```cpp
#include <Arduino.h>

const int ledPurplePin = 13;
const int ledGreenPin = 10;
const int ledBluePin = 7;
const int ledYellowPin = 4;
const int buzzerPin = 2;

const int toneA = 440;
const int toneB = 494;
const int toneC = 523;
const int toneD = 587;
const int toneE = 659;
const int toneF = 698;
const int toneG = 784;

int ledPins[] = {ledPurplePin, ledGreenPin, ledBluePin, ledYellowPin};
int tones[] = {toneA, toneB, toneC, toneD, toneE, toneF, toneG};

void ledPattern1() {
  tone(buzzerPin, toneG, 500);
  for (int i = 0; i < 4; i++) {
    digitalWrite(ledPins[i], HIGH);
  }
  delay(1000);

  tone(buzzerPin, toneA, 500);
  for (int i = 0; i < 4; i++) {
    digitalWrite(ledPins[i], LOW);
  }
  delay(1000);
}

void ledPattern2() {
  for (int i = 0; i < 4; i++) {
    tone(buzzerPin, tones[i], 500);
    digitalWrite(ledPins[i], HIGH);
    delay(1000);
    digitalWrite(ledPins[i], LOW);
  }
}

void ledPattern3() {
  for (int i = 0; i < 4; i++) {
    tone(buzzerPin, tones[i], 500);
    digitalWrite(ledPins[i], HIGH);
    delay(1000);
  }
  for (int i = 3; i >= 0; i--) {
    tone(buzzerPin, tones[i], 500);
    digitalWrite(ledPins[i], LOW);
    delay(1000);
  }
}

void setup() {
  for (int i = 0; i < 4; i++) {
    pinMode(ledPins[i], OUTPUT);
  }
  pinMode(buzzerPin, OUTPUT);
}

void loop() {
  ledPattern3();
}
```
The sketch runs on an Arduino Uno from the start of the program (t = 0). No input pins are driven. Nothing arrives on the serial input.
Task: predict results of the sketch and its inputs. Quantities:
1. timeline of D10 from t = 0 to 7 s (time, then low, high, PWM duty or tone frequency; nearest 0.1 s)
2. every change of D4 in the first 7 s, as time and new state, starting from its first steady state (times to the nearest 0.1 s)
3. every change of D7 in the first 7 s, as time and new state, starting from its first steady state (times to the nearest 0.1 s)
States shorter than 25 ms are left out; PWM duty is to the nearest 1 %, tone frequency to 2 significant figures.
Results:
0 s low; 1 s high; 6 s low
0 s low; 3 s high; 4 s low
0 s low; 2 s high; 5 s low
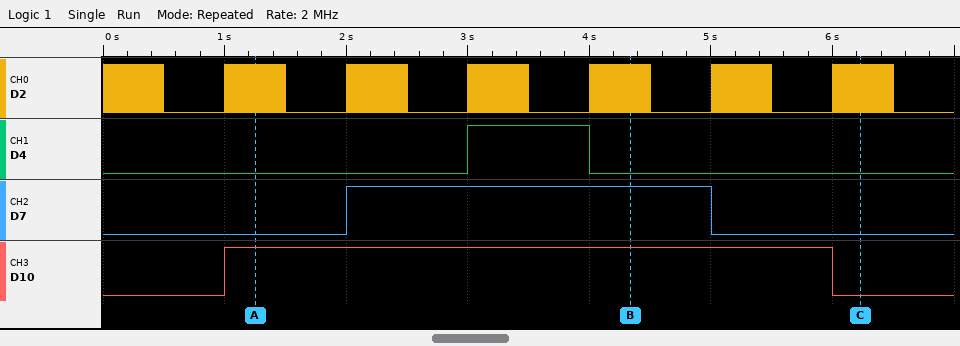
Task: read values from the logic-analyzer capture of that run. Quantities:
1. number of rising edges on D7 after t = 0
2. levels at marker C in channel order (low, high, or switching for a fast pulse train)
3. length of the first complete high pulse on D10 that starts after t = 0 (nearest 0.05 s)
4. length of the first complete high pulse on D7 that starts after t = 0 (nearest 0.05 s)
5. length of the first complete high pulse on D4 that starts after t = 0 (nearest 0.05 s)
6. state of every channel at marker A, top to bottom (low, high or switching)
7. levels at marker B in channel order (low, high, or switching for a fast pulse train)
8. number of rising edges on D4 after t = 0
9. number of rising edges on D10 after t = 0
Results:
1
D2 switching, D4 low, D7 low, D10 low
5.00 s
3.00 s
1.00 s
D2 switching, D4 low, D7 low, D10 high
D2 switching, D4 low, D7 high, D10 high
1
1
